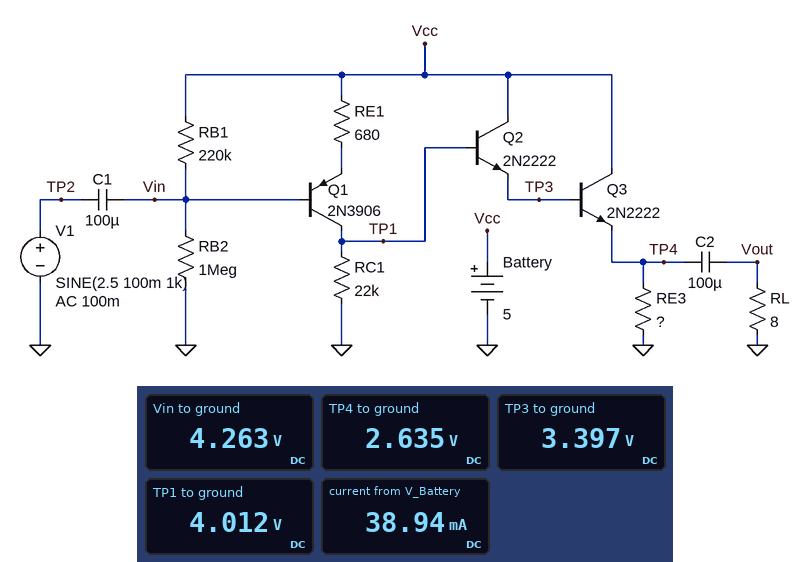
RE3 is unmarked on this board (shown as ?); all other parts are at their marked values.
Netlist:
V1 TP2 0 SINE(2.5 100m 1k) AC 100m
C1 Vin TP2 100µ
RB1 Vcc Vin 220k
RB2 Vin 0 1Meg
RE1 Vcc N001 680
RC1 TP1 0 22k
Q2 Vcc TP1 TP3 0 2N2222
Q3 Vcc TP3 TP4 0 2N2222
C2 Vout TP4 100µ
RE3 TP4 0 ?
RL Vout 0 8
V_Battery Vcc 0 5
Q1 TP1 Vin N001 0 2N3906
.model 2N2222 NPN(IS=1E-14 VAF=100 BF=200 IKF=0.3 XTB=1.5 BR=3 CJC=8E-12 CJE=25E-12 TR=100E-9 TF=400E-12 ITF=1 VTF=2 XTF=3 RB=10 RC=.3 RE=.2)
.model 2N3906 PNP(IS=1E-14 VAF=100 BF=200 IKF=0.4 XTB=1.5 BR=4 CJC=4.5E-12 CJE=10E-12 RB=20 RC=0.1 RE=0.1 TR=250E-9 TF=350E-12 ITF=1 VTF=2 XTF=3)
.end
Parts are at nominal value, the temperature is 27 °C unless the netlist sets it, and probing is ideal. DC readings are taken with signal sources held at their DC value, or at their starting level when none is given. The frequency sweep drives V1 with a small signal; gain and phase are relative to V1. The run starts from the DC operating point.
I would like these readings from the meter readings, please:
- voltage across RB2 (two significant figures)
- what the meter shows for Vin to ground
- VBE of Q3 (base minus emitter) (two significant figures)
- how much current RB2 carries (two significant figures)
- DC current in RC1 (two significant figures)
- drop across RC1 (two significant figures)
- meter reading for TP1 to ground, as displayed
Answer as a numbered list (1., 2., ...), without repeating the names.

1. 4.3 V
2. 4.263 V
3. 760 mV
4. 4.3 µA
5. 180 µA
6. 4.0 V
7. 4.012 V
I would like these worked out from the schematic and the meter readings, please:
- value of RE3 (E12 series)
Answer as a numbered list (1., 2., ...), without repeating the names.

1. 68 Ω
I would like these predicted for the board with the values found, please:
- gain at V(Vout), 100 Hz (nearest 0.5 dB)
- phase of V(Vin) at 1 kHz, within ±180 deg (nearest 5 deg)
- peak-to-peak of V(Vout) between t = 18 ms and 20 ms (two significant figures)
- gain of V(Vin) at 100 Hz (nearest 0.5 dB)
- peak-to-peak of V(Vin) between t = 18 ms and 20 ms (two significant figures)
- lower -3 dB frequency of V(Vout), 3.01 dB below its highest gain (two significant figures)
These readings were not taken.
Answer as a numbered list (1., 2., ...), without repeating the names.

1. 20.5 dB
2. 0 deg
3. 780 mV
4. 0 dB
5. 200 mV
6. 150 Hz
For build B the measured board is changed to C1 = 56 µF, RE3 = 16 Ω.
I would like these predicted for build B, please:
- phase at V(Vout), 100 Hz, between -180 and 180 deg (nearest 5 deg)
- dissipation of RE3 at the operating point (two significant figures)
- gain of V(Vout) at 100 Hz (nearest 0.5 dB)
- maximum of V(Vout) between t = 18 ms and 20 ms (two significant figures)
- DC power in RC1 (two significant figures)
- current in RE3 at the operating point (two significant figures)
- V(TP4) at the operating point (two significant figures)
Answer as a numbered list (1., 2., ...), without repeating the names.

1. -120 deg
2. 370 mW
3. 20.0 dB
4. 950 mV
5. 700 µW
6. 150 mA
7. 2.4 V
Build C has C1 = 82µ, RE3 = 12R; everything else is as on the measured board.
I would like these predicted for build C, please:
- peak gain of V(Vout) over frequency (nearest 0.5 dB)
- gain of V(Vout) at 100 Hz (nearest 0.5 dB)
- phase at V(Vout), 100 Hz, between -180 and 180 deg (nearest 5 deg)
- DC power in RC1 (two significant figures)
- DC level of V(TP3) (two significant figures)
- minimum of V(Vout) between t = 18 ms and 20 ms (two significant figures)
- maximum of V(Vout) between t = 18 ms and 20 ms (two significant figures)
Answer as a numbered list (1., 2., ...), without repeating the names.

1. 25.5 dB
2. 20.0 dB
3. -120 deg
4. 680 µW
5. 3.2 V
6. -960 mV
7. 1.0 V
